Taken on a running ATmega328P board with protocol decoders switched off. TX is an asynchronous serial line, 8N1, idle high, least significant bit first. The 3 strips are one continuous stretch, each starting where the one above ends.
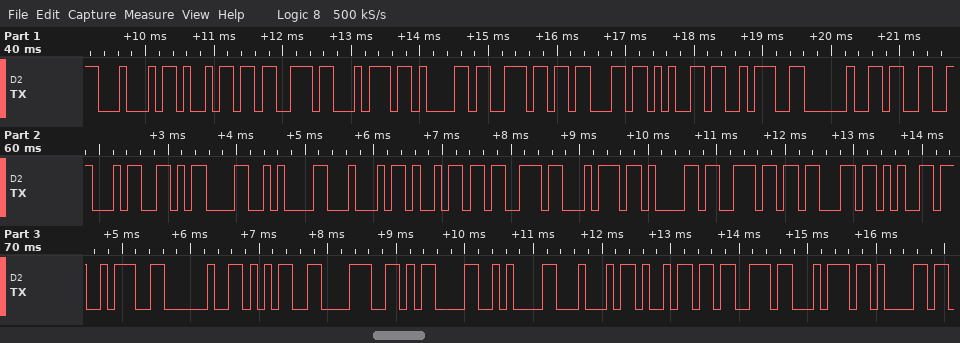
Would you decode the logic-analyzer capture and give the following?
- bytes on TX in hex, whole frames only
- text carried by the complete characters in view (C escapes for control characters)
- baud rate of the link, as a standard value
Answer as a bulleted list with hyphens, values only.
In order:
- 44 69 73 74 61 6E 63 65 3A 20 33 34 0D 0A 44 69 73 74 61 6E 63 65 3A 20 35 38 0D 0A 44 69 73 74 61
- "Distance: 34\r\nDistance: 58\r\nDista"
- 9600 baud
